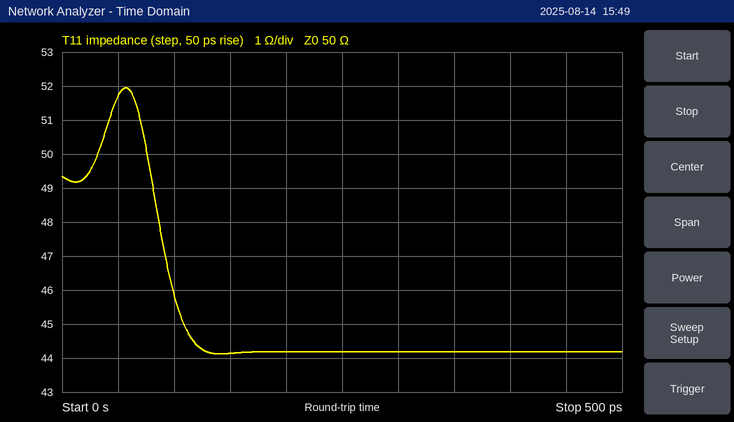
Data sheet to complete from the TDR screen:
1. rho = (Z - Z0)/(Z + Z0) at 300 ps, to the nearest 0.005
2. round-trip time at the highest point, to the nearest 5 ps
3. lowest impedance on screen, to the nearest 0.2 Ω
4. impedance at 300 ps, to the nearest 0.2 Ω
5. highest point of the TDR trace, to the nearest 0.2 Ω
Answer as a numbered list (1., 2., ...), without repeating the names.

1. -0.060
2. 55 ps
3. 44.2 Ω
4. 44.2 Ω
5. 52.0 Ω
